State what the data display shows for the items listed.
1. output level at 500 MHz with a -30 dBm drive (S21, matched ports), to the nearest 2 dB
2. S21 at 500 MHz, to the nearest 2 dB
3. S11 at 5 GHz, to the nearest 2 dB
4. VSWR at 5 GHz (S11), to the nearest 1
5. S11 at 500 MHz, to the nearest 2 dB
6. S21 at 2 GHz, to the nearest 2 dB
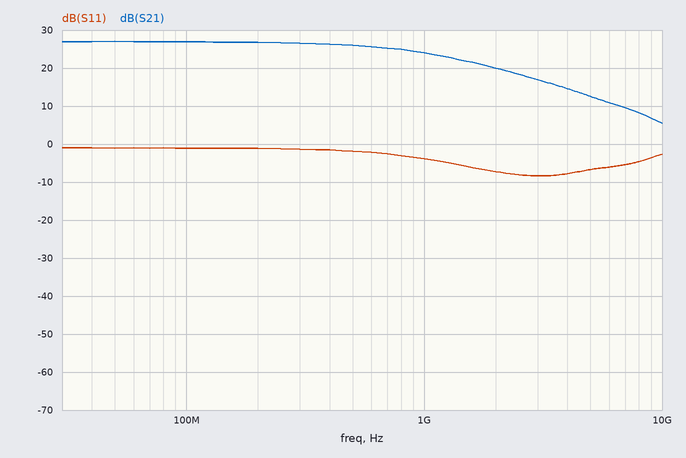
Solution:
-4 dBm
26 dB
-6 dB
3
-2 dB
20 dB
